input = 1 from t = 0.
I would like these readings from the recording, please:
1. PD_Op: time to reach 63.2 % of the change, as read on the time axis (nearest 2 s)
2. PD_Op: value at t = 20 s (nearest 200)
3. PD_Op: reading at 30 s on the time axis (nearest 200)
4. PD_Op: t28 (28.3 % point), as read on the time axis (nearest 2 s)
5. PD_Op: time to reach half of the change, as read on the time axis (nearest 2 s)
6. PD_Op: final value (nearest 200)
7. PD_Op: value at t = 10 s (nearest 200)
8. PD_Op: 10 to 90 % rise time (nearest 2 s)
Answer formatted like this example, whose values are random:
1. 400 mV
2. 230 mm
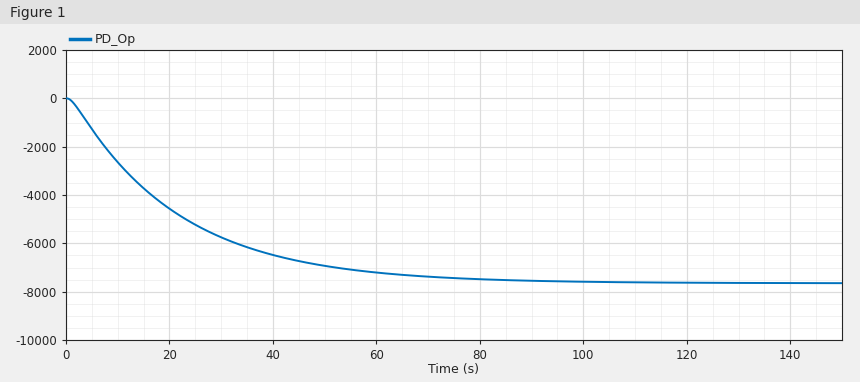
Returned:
1. 22 s
2. -4600
3. -5800
4. 8 s
5. 16 s
6. -7600
7. -2600
8. 46 s
